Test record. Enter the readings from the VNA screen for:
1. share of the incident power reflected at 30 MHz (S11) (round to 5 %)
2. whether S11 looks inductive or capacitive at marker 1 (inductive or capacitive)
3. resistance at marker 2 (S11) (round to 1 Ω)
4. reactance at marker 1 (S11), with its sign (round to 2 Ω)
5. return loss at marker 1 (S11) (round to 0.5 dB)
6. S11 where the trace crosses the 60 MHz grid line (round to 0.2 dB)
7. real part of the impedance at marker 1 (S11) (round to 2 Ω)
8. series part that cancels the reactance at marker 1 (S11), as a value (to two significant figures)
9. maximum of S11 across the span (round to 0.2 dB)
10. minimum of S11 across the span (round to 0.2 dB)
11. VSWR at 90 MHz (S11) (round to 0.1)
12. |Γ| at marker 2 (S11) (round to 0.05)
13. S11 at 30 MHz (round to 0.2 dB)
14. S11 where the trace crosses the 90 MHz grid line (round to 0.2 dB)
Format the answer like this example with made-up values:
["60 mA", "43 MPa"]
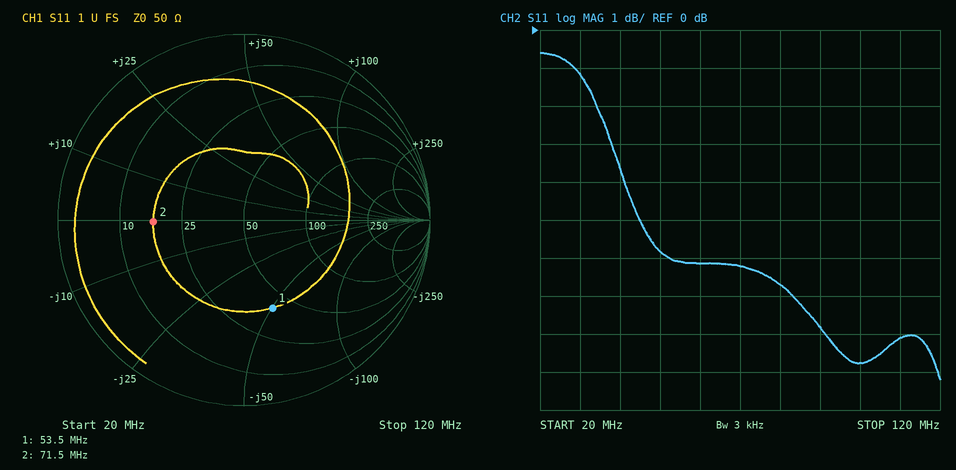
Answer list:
["75 %", "capacitive", "17 Ω", "-50 Ω", "6.0 dB", "-6.2 dB", "40 Ω", "150 nH", "-0.6 dB", "-9.2 dB", "2.4", "0.50", "-1.2 dB", "-7.8 dB"]
